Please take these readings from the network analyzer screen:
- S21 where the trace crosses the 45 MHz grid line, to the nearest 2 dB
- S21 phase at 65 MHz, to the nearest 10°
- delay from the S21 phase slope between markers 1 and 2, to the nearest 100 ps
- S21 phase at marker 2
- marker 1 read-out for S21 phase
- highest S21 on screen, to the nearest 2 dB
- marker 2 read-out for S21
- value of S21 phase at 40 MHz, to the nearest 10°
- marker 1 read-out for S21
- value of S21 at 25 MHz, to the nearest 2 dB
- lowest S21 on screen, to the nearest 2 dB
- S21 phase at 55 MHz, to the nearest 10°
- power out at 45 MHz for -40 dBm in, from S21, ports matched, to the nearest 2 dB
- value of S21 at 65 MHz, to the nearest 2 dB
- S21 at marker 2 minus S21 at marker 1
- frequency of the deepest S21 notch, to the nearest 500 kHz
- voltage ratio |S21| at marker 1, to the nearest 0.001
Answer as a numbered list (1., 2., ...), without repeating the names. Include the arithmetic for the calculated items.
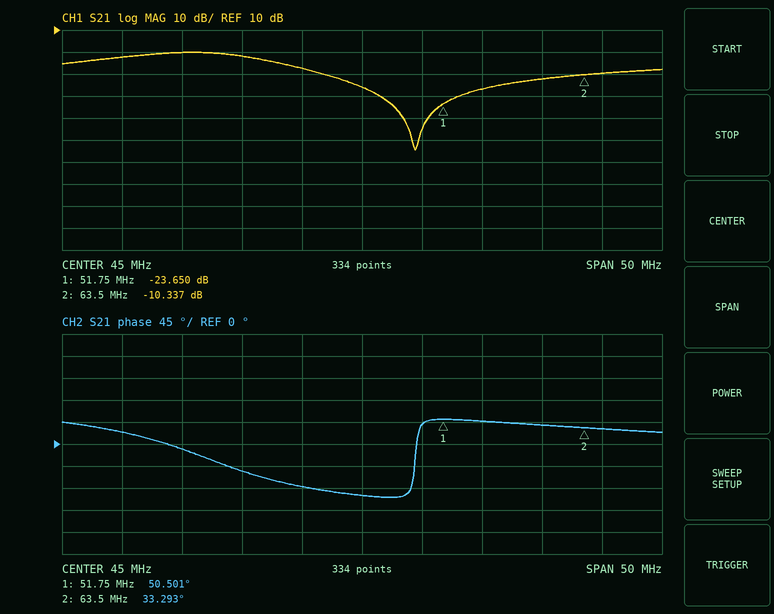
1. -16 dB
2. 30°
3. −(33.293° − (50.501°))/(360° × 11.75 MHz) ≈ 4.1 ns
4. 33.293°
5. 50.501°
6. 0 dB
7. -10.337 dB
8. -90°
9. -23.650 dB
10. -2 dB
11. -44 dB
12. 50°
13. -40 dBm + (-16 dB) = -56 dBm
14. -10 dB
15. -10.337 − (-23.65) = 13.313 dB
16. 49.5 MHz
17. 10^(-23.65/20) ≈ 0.066
